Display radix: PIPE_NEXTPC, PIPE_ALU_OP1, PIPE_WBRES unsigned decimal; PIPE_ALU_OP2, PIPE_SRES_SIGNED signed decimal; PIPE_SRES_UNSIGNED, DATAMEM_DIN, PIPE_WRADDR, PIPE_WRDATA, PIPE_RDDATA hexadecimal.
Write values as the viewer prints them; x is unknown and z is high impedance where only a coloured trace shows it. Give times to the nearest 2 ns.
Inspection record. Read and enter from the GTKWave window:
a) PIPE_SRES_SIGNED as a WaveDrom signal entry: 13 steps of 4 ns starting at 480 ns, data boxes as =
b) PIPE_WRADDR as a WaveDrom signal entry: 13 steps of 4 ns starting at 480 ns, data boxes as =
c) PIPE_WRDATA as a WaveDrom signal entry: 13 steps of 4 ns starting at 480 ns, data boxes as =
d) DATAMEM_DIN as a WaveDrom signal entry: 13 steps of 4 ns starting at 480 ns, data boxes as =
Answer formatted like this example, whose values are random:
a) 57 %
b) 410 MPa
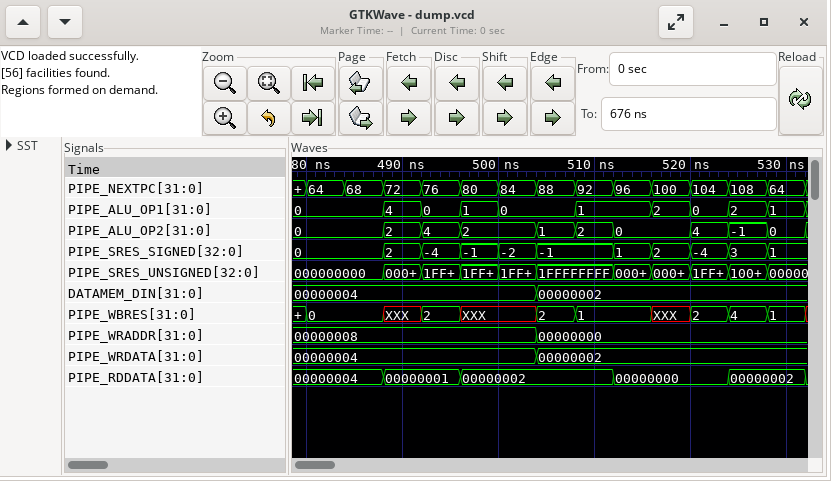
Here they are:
a) {name: 'PIPE_SRES_SIGNED', wave: '=.=====.=====', data: '0 2 -4 -1 -2 -1 1 2 -4 3 1'}
b) {name: 'PIPE_WRADDR', wave: '=.....=......', data: '00000008 00000000'}
c) {name: 'PIPE_WRDATA', wave: '=.....=......', data: '00000004 00000002'}
d) {name: 'DATAMEM_DIN', wave: '=.....=......', data: '00000004 00000002'}
